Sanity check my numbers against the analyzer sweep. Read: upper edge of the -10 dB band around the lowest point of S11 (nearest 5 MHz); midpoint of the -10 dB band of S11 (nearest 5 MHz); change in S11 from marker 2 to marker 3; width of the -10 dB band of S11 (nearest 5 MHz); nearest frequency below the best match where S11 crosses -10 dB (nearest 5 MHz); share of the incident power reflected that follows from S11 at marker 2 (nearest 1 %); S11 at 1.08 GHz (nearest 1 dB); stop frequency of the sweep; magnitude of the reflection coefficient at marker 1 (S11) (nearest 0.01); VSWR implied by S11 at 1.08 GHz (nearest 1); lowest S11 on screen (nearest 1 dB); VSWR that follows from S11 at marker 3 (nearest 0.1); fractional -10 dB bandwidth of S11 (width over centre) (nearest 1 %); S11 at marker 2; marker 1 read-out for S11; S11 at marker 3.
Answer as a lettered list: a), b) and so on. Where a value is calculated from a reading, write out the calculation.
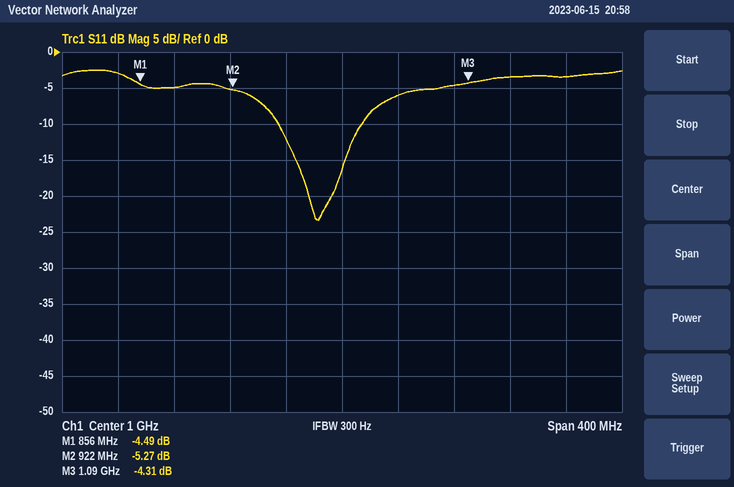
a) 1.015 GHz
b) 985 MHz
c) -4.31 − (-5.27) = 0.96 dB
d) 1.015 GHz − 955 MHz = 60 MHz
e) 955 MHz
f) 10^(-5.27/10) ≈ 30 %
g) -5 dB
h) 1.2 GHz
i) 10^(-4.49/20) ≈ 0.60
j) |Γ| = 10^(-5/20) = 0.5623; VSWR = (1 + 0.5623)/(1 − 0.5623) ≈ 4
k) -23 dB
l) (1 + 0.6088)/(1 − 0.6088) ≈ 4.1
m) 60 MHz / 985 MHz ≈ 6 %
n) -5.27 dB
o) -4.49 dB
p) -4.31 dB
